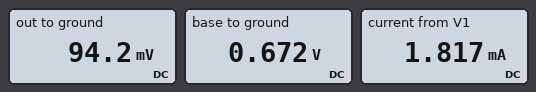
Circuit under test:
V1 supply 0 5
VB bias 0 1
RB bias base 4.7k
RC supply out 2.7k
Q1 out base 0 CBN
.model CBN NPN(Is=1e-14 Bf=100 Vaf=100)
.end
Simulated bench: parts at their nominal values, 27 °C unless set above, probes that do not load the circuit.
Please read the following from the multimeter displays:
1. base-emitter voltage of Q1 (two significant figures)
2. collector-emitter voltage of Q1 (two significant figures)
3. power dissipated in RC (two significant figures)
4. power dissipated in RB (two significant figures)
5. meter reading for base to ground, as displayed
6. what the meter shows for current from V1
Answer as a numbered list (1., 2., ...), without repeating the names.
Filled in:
1. 670 mV
2. 94 mV
3. 8.9 mW
4. 23 µW
5. 0.672 V
6. 1.817 mA
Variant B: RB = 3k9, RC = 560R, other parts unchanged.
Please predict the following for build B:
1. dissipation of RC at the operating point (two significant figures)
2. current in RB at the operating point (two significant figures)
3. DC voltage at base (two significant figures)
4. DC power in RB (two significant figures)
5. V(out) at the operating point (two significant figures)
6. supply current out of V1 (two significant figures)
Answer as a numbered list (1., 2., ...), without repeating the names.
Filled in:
1. 32 mW
2. 75 µA
3. 710 mV
4. 22 µW
5. 790 mV
6. 7.5 mA
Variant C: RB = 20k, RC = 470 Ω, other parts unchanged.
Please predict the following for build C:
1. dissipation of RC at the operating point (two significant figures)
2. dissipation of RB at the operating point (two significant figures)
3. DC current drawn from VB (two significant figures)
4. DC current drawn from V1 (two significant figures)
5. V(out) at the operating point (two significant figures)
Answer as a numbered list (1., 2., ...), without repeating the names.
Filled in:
1. 1.4 mW
2. 5.5 µW
3. 17 µA
4. 1.7 mA
5. 4.2 V
